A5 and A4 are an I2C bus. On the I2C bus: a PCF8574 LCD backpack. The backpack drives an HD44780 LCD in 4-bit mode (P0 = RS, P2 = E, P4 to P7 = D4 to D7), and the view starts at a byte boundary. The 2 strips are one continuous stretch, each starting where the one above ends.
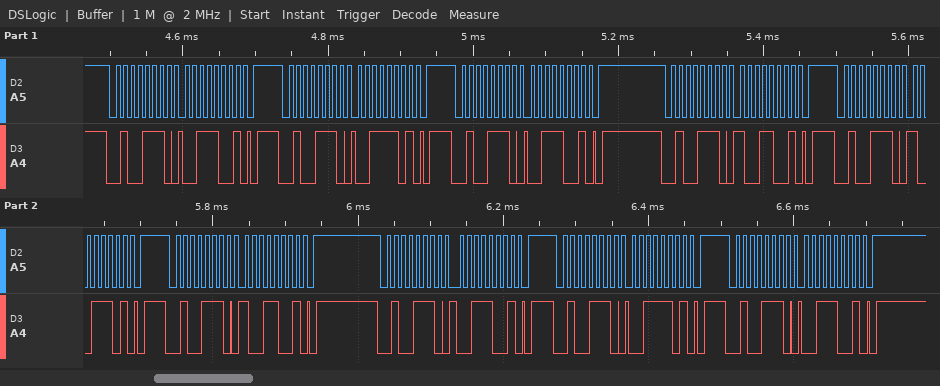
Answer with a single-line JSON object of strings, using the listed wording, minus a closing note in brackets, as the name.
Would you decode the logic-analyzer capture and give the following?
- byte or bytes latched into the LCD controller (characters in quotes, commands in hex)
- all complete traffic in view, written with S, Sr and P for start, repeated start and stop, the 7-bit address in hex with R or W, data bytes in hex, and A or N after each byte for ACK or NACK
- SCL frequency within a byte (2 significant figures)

{"byte or bytes latched into the LCD controller": "'9'", "all complete traffic in view, written with S, Sr and P for start, repeated start and stop, the 7-bit address in hex with R or W, data bytes in hex, and A or N after each byte for ACK or NACK": "S 27W A 39 A P S 27W A 3D A P S 27W A 39 A P S 27W A 99 A P S 27W A 9D A P S 27W A 99 A P S 27W A 39 A P S 27W A 3D A P S 27W A 39 A P", "SCL frequency within a byte": "100 kHz"}
